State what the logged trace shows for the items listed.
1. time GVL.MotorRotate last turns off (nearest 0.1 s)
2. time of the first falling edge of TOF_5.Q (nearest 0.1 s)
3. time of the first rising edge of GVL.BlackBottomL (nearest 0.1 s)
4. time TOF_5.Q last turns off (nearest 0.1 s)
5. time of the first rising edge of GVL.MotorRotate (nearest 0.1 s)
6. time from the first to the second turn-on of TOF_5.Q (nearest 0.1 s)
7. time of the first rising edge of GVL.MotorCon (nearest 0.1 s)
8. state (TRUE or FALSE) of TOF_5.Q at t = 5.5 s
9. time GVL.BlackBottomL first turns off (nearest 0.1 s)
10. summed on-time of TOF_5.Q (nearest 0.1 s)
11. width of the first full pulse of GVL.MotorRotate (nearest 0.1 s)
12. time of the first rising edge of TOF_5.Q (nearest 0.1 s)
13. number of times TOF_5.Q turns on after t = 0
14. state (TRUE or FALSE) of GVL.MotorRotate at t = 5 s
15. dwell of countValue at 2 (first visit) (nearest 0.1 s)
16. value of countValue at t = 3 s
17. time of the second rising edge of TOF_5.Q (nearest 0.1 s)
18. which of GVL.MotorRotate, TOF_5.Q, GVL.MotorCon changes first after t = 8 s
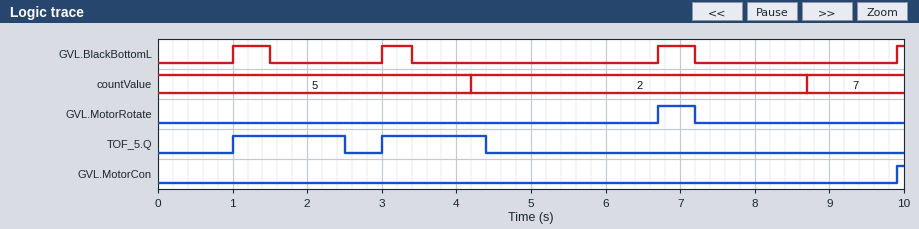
7.2 s
2.5 s
1.0 s
4.4 s
6.7 s
2.0 s
9.9 s
FALSE
1.5 s
2.9 s
0.5 s
1.0 s
2
FALSE
4.5 s
5
3.0 s
GVL.MotorCon
